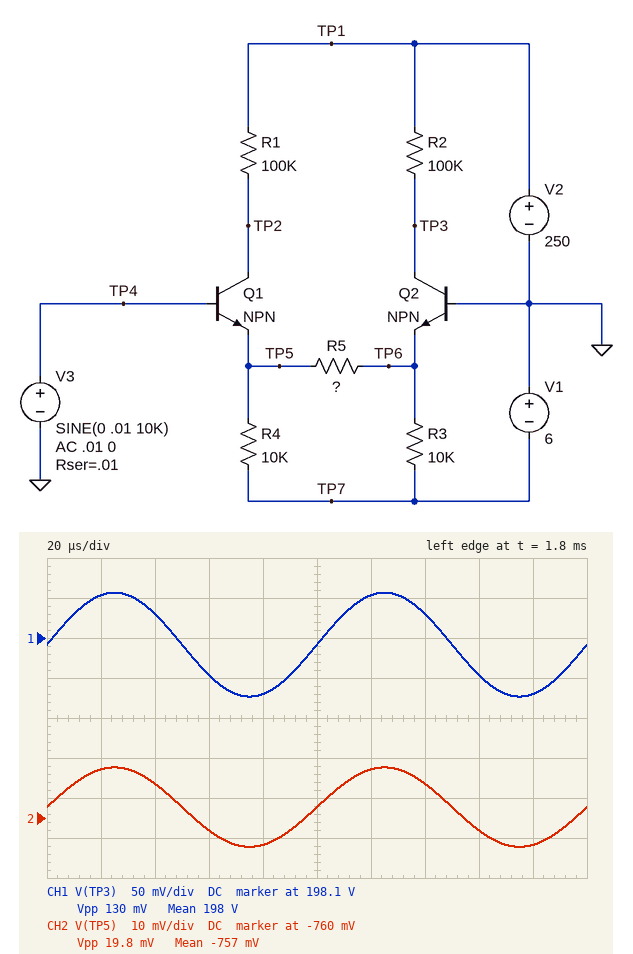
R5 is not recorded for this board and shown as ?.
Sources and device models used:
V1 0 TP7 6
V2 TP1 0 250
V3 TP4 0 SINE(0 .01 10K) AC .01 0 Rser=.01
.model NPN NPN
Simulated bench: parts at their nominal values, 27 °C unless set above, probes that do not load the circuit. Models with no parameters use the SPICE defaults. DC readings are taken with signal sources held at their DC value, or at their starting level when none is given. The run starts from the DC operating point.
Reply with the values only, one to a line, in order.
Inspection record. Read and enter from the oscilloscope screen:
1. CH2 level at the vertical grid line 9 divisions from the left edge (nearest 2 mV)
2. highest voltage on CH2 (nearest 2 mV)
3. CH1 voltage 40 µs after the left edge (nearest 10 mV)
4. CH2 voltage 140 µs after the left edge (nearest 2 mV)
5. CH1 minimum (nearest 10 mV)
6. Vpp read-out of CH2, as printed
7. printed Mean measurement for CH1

-766 mV
-748 mV
198.13 V
-752 mV
198.03 V
19.8 mV
198 V
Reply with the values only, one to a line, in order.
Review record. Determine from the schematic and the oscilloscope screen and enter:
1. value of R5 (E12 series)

15 kΩ
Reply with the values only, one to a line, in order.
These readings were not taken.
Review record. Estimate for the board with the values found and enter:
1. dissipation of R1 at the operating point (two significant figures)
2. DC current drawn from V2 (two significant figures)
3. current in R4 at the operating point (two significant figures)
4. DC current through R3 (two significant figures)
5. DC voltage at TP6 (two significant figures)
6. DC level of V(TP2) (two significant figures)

27 mW
1.0 mA
520 µA
520 µA
-760 mV
200 V
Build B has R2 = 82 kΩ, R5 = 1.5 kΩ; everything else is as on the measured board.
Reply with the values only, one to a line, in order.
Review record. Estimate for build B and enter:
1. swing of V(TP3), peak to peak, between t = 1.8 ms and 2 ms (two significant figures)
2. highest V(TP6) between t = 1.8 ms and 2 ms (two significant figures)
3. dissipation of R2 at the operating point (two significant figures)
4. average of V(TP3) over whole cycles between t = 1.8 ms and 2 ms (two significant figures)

1.0 V
-760 mV
22 mW
210 V
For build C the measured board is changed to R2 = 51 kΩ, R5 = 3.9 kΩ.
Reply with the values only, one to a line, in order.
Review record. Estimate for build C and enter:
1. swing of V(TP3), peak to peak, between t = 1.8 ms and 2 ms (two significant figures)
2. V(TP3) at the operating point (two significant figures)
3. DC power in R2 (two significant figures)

250 mV
220 V
14 mW
